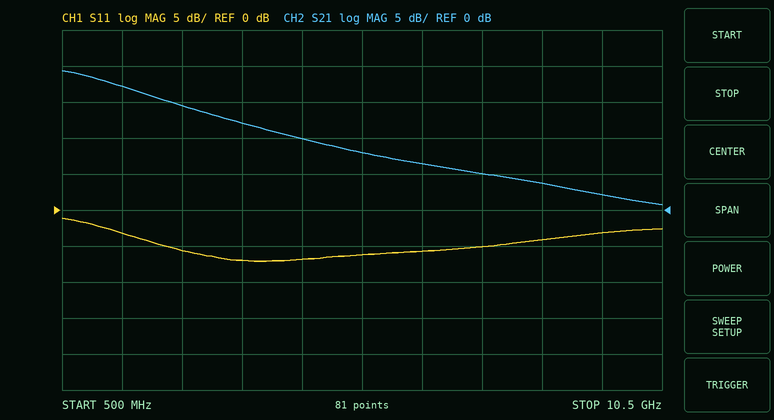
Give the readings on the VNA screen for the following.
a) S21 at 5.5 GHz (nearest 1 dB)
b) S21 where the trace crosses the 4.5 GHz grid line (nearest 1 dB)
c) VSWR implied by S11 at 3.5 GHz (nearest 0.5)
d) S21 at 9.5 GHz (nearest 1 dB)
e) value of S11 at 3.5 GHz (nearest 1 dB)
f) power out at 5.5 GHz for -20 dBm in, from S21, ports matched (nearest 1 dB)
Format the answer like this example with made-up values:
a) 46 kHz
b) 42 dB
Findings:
a) 8 dB
b) 10 dB
c) 2.5
d) 2 dB
e) -7 dB
f) -12 dBm
